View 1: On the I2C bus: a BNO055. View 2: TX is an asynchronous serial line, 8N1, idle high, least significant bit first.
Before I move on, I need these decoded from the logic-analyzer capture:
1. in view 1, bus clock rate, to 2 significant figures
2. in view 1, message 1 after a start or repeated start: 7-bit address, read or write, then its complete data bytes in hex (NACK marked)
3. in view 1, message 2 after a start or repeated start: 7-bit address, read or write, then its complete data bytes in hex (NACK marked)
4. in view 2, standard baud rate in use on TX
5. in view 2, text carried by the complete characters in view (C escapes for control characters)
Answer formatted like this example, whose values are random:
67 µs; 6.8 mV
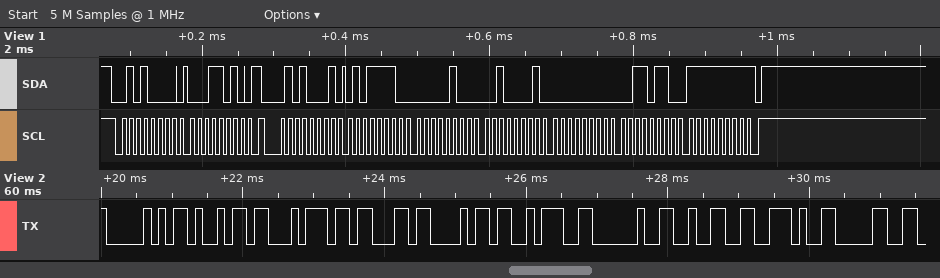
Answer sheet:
100 kHz; 0x28 write: 1A; 0x28 read: 5E 04 21 00 36 FF NACK; 9600 baud; "Pitch: 2.0"
